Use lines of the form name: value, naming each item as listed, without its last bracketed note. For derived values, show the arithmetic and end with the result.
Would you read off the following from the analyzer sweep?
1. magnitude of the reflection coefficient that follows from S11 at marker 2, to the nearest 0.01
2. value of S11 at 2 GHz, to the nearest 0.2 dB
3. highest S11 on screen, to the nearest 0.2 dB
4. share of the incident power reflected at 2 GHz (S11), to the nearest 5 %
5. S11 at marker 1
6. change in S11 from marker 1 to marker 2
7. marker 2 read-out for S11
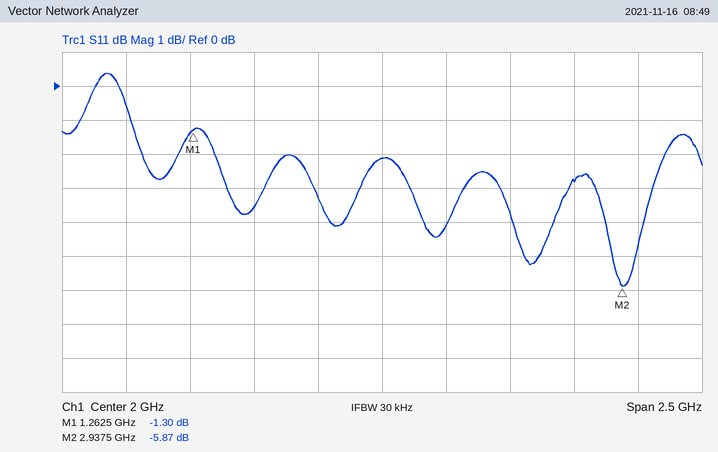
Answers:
magnitude of the reflection coefficient that follows from S11 at marker 2, to the nearest 0.01: 10^(-5.87/20) ≈ 0.51
value of S11 at 2 GHz, to the nearest 0.2 dB: -2.2 dB
highest S11 on screen, to the nearest 0.2 dB: 0.4 dB
share of the incident power reflected at 2 GHz (S11), to the nearest 5 %: 10^(-2.2/10) ≈ 60 %
S11 at marker 1: -1.30 dB
change in S11 from marker 1 to marker 2: -5.87 − (-1.3) = -4.57 dB
marker 2 read-out for S11: -5.87 dB
